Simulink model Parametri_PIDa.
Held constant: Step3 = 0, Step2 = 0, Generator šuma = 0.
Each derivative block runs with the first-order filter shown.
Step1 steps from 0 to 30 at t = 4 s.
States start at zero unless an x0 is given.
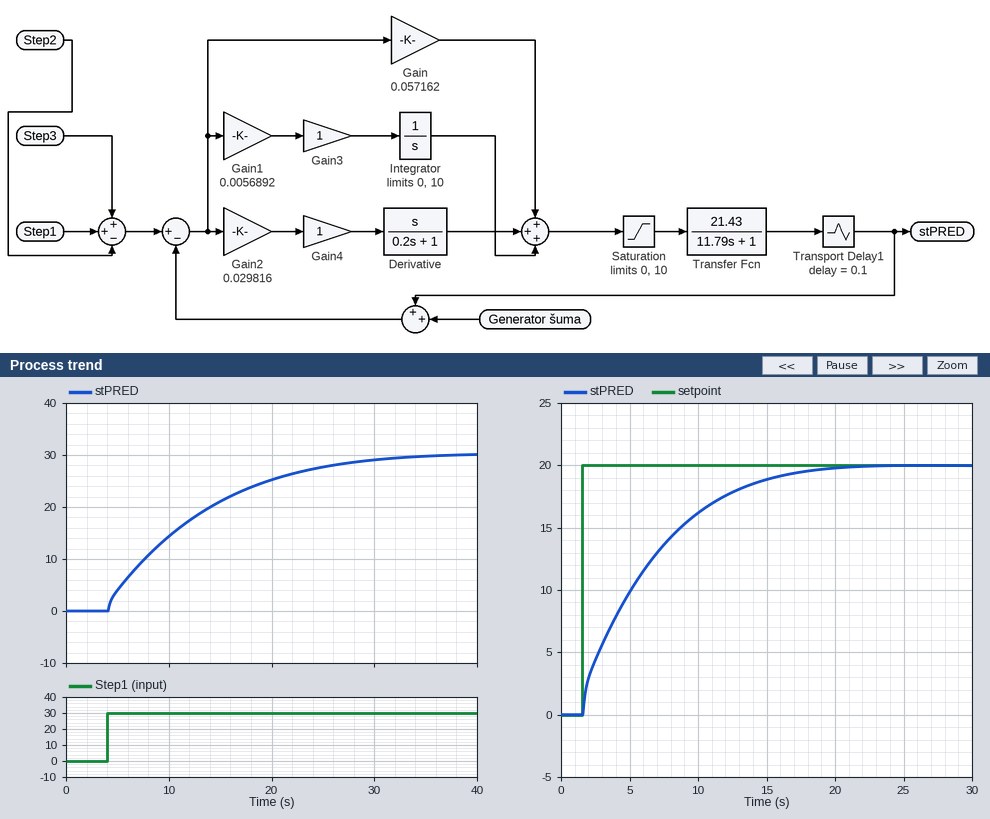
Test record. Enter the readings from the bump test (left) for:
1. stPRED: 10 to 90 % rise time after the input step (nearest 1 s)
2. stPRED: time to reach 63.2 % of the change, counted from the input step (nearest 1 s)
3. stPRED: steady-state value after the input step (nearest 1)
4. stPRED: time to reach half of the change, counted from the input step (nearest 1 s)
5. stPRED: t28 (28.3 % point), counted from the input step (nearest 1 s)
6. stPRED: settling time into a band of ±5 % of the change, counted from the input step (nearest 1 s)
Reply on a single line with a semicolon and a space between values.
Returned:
19 s; 9 s; 30; 6 s; 3 s; 24 s
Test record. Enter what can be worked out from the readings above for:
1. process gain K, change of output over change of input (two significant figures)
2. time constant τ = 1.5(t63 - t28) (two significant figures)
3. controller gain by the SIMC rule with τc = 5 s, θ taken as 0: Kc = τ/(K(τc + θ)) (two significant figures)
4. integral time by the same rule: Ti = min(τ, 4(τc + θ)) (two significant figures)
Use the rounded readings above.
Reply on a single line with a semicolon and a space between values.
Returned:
1.0; 9.0 s; 1.8; 9.0 s
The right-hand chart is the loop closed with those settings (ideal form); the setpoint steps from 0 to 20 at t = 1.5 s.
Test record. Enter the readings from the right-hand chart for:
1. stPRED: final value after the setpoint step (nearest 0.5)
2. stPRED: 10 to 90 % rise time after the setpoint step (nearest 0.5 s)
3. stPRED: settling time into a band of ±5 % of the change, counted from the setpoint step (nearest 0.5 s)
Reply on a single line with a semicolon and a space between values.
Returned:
20.0; 11.0 s; 14.0 s
